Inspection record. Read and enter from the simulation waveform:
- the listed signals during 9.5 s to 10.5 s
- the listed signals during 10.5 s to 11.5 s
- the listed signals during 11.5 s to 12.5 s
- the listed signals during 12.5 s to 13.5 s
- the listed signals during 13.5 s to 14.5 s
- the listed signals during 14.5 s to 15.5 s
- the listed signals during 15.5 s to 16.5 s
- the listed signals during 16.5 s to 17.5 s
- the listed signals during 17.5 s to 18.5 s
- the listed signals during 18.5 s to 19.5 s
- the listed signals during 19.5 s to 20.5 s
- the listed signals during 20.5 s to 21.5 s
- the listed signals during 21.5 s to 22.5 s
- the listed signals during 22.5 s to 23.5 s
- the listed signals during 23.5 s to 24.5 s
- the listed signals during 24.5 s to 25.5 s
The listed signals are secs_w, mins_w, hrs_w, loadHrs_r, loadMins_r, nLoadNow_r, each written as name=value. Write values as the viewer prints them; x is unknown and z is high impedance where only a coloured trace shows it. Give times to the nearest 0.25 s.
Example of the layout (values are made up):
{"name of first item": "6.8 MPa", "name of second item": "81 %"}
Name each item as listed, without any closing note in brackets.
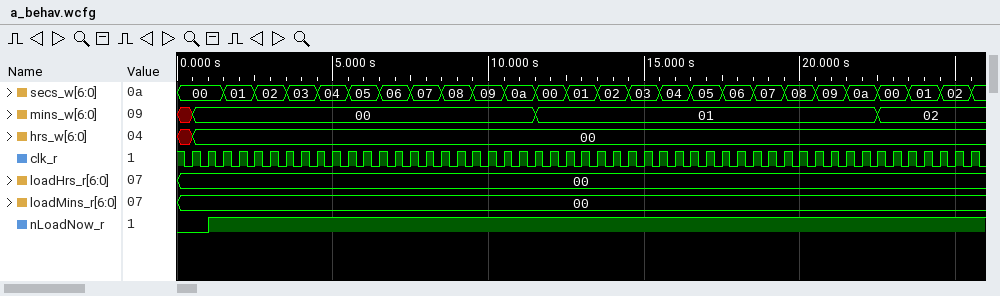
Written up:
{"the listed signals during 9.5 s to 10.5 s": "secs_w=09, mins_w=00, hrs_w=00, loadHrs_r=00, loadMins_r=00, nLoadNow_r=1", "the listed signals during 10.5 s to 11.5 s": "secs_w=0a, mins_w=00, hrs_w=00, loadHrs_r=00, loadMins_r=00, nLoadNow_r=1", "the listed signals during 11.5 s to 12.5 s": "secs_w=00, mins_w=01, hrs_w=00, loadHrs_r=00, loadMins_r=00, nLoadNow_r=1", "the listed signals during 12.5 s to 13.5 s": "secs_w=01, mins_w=01, hrs_w=00, loadHrs_r=00, loadMins_r=00, nLoadNow_r=1", "the listed signals during 13.5 s to 14.5 s": "secs_w=02, mins_w=01, hrs_w=00, loadHrs_r=00, loadMins_r=00, nLoadNow_r=1", "the listed signals during 14.5 s to 15.5 s": "secs_w=03, mins_w=01, hrs_w=00, loadHrs_r=00, loadMins_r=00, nLoadNow_r=1", "the listed signals during 15.5 s to 16.5 s": "secs_w=04, mins_w=01, hrs_w=00, loadHrs_r=00, loadMins_r=00, nLoadNow_r=1", "the listed signals during 16.5 s to 17.5 s": "secs_w=05, mins_w=01, hrs_w=00, loadHrs_r=00, loadMins_r=00, nLoadNow_r=1", "the listed signals during 17.5 s to 18.5 s": "secs_w=06, mins_w=01, hrs_w=00, loadHrs_r=00, loadMins_r=00, nLoadNow_r=1", "the listed signals during 18.5 s to 19.5 s": "secs_w=07, mins_w=01, hrs_w=00, loadHrs_r=00, loadMins_r=00, nLoadNow_r=1", "the listed signals during 19.5 s to 20.5 s": "secs_w=08, mins_w=01, hrs_w=00, loadHrs_r=00, loadMins_r=00, nLoadNow_r=1", "the listed signals during 20.5 s to 21.5 s": "secs_w=09, mins_w=01, hrs_w=00, loadHrs_r=00, loadMins_r=00, nLoadNow_r=1", "the listed signals during 21.5 s to 22.5 s": "secs_w=0a, mins_w=01, hrs_w=00, loadHrs_r=00, loadMins_r=00, nLoadNow_r=1", "the listed signals during 22.5 s to 23.5 s": "secs_w=00, mins_w=02, hrs_w=00, loadHrs_r=00, loadMins_r=00, nLoadNow_r=1", "the listed signals during 23.5 s to 24.5 s": "secs_w=01, mins_w=02, hrs_w=00, loadHrs_r=00, loadMins_r=00, nLoadNow_r=1", "the listed signals during 24.5 s to 25.5 s": "secs_w=02, mins_w=02, hrs_w=00, loadHrs_r=00, loadMins_r=00, nLoadNow_r=1"}
